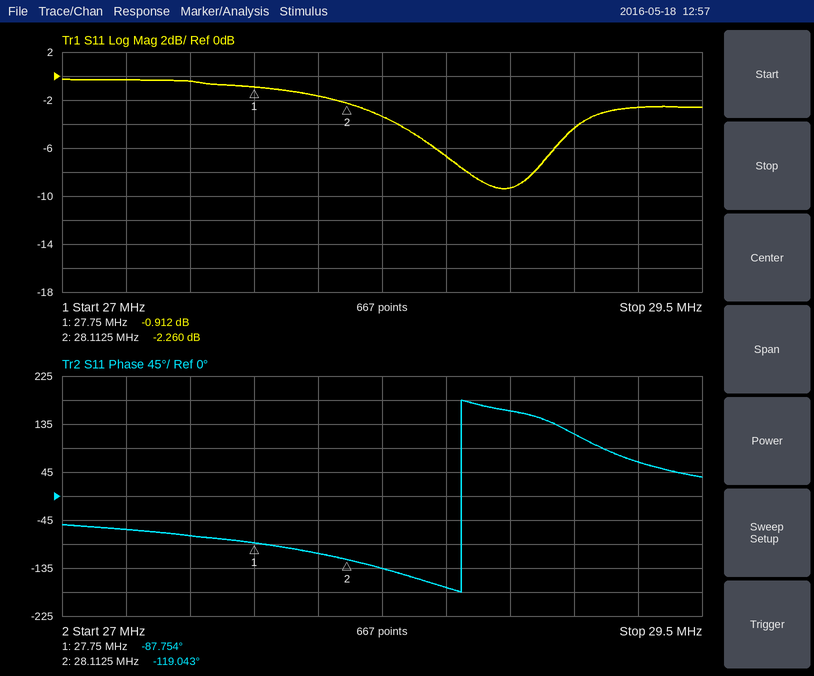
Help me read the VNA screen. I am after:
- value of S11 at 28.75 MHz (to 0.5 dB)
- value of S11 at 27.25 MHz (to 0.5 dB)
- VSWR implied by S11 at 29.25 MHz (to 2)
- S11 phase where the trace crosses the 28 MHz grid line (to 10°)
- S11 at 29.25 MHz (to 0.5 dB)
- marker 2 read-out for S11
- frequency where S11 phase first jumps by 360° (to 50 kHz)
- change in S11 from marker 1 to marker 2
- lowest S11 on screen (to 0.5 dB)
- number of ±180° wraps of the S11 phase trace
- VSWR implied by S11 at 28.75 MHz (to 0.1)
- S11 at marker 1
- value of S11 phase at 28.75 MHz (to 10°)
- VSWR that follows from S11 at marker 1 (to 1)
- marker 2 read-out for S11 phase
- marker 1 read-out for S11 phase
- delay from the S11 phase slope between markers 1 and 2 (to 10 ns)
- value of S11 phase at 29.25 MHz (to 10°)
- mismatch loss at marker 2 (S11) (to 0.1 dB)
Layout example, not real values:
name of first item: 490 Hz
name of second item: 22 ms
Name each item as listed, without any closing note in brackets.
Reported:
value of S11 at 28.75 MHz: -9.5 dB
value of S11 at 27.25 MHz: -0.5 dB
VSWR implied by S11 at 29.25 MHz: 6
S11 phase where the trace crosses the 28 MHz grid line: -110°
S11 at 29.25 MHz: -2.5 dB
marker 2 read-out for S11: -2.260 dB
frequency where S11 phase first jumps by 360°: 28.55 MHz
change in S11 from marker 1 to marker 2: -1.348 dB
lowest S11 on screen: -9.5 dB
number of ±180° wraps of the S11 phase trace: 1
VSWR implied by S11 at 28.75 MHz: 2.0
S11 at marker 1: -0.912 dB
value of S11 phase at 28.75 MHz: 160°
VSWR that follows from S11 at marker 1: 19
marker 2 read-out for S11 phase: -119.043°
marker 1 read-out for S11 phase: -87.754°
delay from the S11 phase slope between markers 1 and 2: 240 ns
value of S11 phase at 29.25 MHz: 60°
mismatch loss at marker 2 (S11): 3.9 dB
